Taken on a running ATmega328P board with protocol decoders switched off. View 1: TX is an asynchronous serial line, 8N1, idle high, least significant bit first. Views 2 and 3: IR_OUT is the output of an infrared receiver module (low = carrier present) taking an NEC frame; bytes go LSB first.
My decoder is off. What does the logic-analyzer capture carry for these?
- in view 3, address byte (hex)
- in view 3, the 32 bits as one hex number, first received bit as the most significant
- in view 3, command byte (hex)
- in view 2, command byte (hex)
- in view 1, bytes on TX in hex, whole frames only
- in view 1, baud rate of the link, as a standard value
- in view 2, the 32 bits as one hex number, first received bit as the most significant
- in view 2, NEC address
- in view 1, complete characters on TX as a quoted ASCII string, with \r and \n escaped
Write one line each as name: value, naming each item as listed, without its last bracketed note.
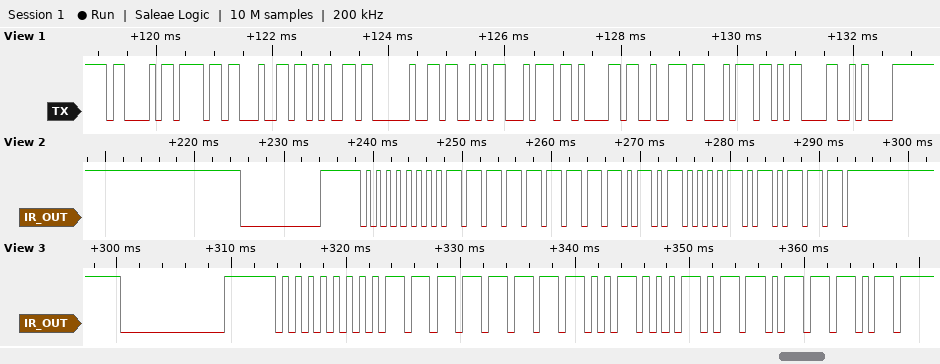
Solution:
in view 3, address byte: 0x00
in view 3, the 32 bits as one hex number, first received bit as the most significant: 0x00FF22DD
in view 3, command byte: 0x44
in view 2, command byte: 0x15
in view 1, bytes on TX in hex, whole frames only: 0x43 0x6F 0x64 0x65 0x20 0x53 0x74 0x61 0x72 0x74 0x0D 0x0A
in view 1, baud rate of the link, as a standard value: 9600 baud
in view 2, the 32 bits as one hex number, first received bit as the most significant: 0x00FFA857
in view 2, NEC address: 0x00
in view 1, complete characters on TX as a quoted ASCII string, with \r and \n escaped: "Code Start\r\n"
